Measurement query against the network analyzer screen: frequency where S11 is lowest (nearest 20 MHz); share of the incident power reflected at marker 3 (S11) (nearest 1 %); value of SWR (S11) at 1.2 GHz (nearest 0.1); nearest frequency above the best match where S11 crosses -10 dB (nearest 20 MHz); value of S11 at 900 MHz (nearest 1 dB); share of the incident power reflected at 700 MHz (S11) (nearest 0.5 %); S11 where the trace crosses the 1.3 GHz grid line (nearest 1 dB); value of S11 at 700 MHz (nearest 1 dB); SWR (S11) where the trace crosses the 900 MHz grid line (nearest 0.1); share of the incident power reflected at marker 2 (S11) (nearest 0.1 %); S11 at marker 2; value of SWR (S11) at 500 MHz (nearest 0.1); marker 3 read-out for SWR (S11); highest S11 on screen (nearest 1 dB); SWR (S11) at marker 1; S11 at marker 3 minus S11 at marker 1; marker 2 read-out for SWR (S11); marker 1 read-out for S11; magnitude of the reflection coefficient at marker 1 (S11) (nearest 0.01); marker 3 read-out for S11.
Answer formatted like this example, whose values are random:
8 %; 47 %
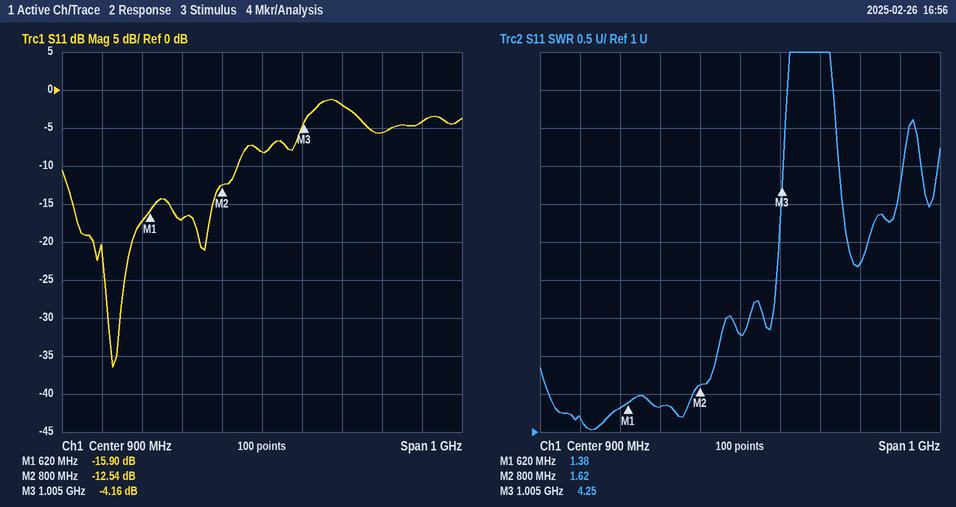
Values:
520 MHz; 38 %; 3.2; 840 MHz; -8 dB; 2.0 %; -4 dB; -17 dB; 2.3; 5.6 %; -12.54 dB; 1.2; 4.25; -1 dB; 1.38; 11.74 dB; 1.62; -15.90 dB; 0.16; -4.16 dB
